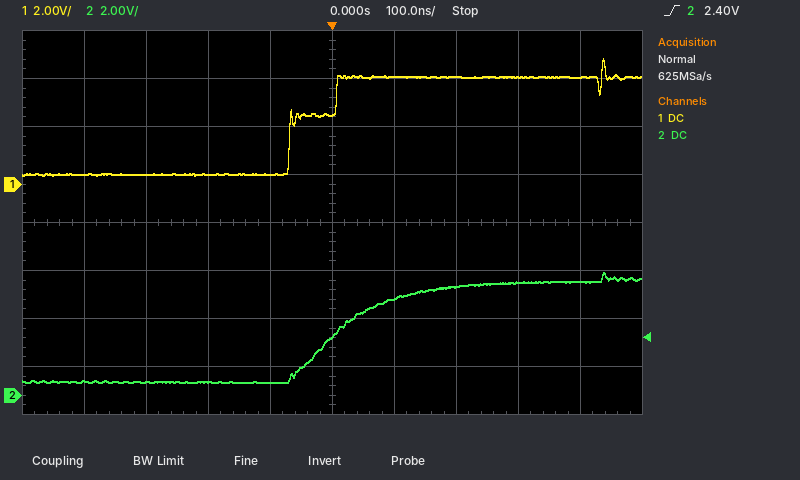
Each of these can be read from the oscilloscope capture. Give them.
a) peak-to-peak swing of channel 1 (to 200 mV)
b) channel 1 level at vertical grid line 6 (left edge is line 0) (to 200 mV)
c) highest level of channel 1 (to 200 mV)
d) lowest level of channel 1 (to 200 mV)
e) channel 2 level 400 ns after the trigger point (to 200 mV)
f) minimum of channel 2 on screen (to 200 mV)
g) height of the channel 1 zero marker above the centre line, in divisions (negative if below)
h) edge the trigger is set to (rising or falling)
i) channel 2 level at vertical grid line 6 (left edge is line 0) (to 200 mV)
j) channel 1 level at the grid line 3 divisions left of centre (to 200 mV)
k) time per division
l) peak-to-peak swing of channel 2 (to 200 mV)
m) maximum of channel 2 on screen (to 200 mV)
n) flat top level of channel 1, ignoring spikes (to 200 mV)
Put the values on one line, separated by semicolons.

4.8 V; 4.4 V; 5.2 V; 400 mV; 4.8 V; 600 mV; +0.8 div; rising; 4.0 V; 400 mV; 100 ns; 4.6 V; 5.2 V; 4.4 V
